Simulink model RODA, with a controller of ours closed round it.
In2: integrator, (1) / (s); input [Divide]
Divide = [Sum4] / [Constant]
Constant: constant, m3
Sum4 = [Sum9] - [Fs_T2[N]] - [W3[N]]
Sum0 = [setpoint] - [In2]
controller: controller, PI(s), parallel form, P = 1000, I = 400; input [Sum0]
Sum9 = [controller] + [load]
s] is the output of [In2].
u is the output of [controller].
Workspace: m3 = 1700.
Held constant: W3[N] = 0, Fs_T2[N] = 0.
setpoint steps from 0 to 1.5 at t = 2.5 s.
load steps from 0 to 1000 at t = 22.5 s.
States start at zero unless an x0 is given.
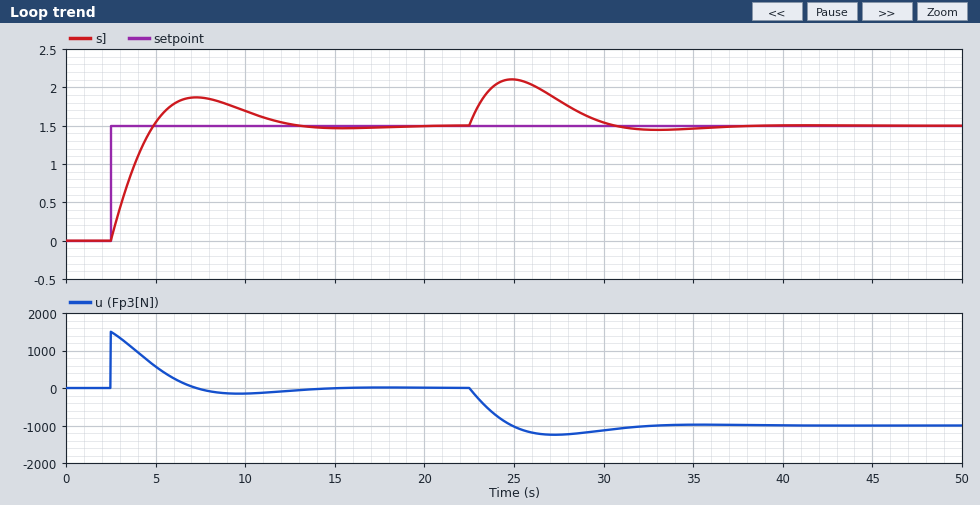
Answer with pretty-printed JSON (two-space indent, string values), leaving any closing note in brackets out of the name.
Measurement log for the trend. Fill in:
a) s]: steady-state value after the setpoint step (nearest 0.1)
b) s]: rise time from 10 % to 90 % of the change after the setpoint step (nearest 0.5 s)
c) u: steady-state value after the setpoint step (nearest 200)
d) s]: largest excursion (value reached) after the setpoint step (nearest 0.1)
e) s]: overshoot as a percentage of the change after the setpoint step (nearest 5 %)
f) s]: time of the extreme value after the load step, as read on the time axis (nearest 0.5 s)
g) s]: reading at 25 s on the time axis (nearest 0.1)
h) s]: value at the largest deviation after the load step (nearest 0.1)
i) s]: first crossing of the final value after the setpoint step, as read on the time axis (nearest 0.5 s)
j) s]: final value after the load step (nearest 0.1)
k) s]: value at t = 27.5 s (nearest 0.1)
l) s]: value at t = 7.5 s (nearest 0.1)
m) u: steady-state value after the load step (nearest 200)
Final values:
{
  "s]: steady-state value after the setpoint step": "1.5",
  "s]: rise time from 10 % to 90 % of the change after the setpoint step": "2.0 s",
  "u: steady-state value after the setpoint step": "0",
  "s]: largest excursion (value reached) after the setpoint step": "1.9",
  "s]: overshoot as a percentage of the change after the setpoint step": "25 %",
  "s]: time of the extreme value after the load step, as read on the time axis": "25.0 s",
  "s]: reading at 25 s on the time axis": "2.1",
  "s]: value at the largest deviation after the load step": "2.1",
  "s]: first crossing of the final value after the setpoint step, as read on the time axis": "5.0 s",
  "s]: final value after the load step": "1.5",
  "s]: value at t = 27.5 s": "1.8",
  "s]: value at t = 7.5 s": "1.9",
  "u: steady-state value after the load step": "-1000"
}
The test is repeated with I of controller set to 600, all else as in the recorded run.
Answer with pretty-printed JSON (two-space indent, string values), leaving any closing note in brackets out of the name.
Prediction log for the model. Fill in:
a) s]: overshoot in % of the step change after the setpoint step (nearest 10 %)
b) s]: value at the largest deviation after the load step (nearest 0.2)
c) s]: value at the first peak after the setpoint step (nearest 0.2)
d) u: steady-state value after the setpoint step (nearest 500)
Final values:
{
  "s]: overshoot in % of the step change after the setpoint step": "30 %",
  "s]: value at the largest deviation after the load step": "2.0",
  "s]: value at the first peak after the setpoint step": "2.0",
  "u: steady-state value after the setpoint step": "0"
}
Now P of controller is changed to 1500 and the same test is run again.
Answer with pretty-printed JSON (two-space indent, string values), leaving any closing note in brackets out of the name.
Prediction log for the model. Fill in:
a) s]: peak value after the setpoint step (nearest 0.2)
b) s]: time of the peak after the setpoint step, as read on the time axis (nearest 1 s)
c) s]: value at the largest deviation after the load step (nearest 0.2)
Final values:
{
  "s]: peak value after the setpoint step": "1.8",
  "s]: time of the peak after the setpoint step, as read on the time axis": "7 s",
  "s]: value at the largest deviation after the load step": "2.0"
}
